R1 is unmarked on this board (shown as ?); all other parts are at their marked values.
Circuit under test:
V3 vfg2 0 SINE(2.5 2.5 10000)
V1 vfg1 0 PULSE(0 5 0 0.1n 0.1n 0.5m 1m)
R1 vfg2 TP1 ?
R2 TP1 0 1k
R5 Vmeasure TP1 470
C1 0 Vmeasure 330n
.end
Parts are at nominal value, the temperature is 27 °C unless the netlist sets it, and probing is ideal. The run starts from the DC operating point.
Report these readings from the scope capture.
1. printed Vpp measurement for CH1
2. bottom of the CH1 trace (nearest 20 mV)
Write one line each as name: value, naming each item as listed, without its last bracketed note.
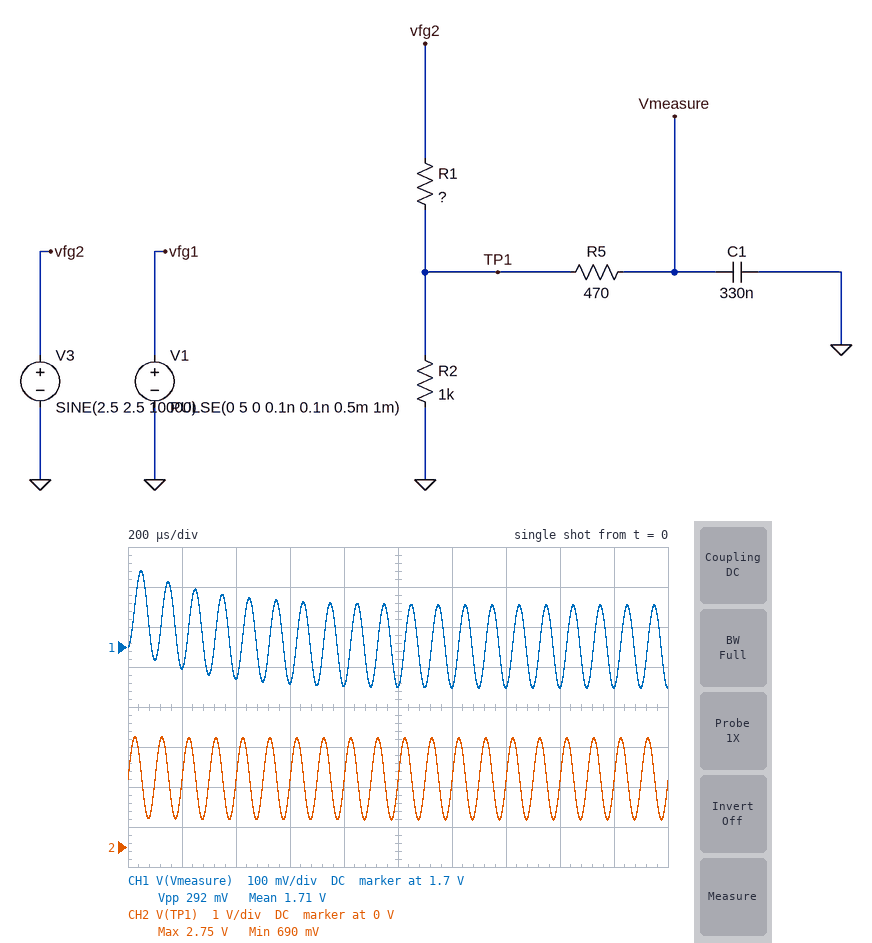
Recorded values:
printed Vpp measurement for CH1: 292 mV
bottom of the CH1 trace: 1.60 V
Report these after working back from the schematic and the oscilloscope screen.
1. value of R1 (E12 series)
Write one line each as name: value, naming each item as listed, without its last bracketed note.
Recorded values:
value of R1: 470 Ω
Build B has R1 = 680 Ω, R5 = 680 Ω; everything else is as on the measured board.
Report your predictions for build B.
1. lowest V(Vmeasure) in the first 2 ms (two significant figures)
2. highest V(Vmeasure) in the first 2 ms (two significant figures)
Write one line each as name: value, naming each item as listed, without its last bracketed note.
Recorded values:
lowest V(Vmeasure) in the first 2 ms: 1.4 V
highest V(Vmeasure) in the first 2 ms: 1.6 V
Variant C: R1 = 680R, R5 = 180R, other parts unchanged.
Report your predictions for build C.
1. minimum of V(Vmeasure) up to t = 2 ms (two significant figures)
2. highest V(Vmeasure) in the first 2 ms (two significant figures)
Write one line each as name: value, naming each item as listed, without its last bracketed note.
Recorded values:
minimum of V(Vmeasure) up to t = 2 ms: 1.4 V
highest V(Vmeasure) in the first 2 ms: 1.7 V
